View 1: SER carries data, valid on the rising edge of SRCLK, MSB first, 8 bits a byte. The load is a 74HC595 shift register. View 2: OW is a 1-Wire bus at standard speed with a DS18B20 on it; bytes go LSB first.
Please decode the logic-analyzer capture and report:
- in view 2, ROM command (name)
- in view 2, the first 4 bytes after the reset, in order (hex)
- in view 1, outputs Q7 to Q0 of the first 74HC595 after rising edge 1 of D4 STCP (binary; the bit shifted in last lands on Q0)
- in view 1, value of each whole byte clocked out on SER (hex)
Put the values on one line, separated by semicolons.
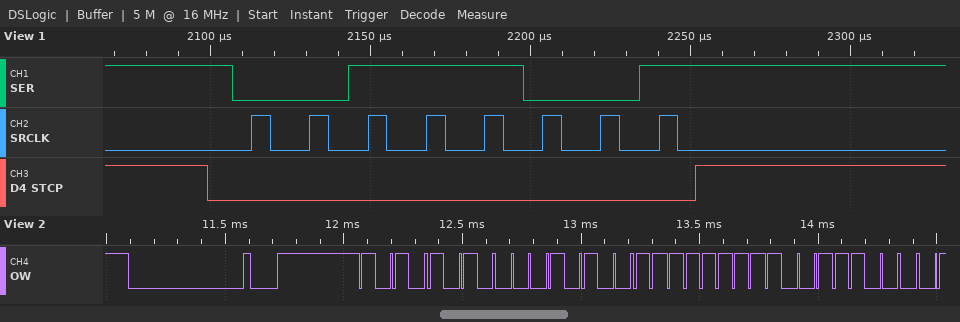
Match ROM; 55 28 FF 39; 00111001; 39
